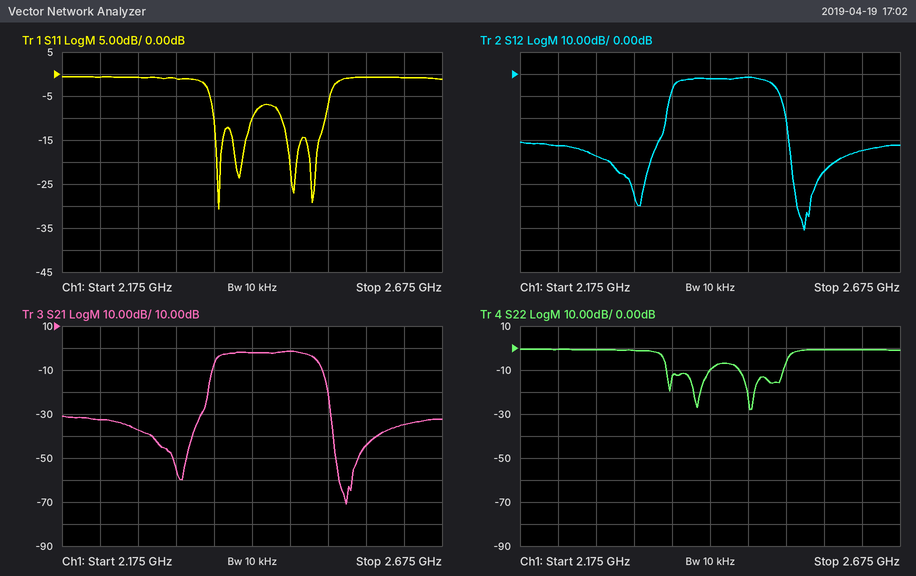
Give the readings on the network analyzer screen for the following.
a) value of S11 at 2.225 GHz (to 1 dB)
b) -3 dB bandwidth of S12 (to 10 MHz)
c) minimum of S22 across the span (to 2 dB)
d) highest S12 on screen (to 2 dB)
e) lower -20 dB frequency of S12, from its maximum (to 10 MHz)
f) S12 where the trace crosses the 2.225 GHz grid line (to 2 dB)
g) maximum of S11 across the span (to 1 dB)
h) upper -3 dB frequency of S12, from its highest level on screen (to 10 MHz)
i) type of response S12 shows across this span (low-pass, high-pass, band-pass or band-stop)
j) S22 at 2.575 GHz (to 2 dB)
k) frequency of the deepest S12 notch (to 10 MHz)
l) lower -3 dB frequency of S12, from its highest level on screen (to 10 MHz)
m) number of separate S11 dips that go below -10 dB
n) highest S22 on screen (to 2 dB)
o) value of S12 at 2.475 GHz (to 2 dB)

-1 dB
130 MHz
-28 dB
-2 dB
2.37 GHz
-32 dB
-1 dB
2.51 GHz
band-pass
0 dB
2.55 GHz
2.38 GHz
4
0 dB
-2 dB
